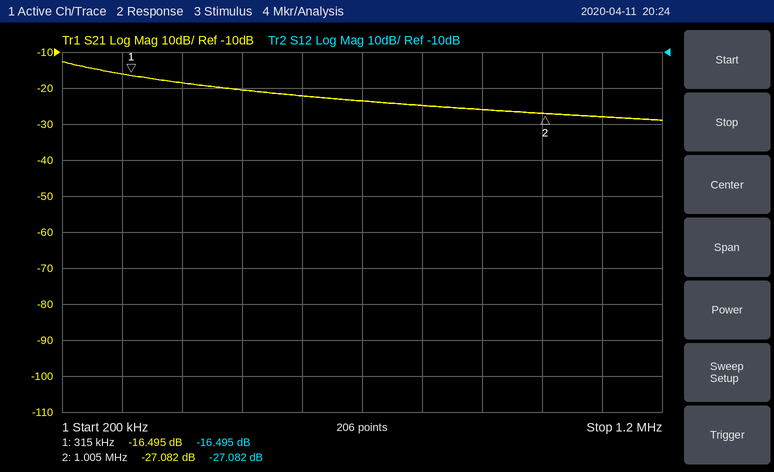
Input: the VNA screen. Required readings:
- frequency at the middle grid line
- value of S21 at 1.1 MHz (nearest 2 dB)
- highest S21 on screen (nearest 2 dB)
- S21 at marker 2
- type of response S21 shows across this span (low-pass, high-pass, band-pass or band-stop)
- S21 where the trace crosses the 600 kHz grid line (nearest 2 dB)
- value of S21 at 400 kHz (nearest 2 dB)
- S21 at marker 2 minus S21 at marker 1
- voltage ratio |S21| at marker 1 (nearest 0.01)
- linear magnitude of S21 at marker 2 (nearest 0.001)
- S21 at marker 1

700 kHz
-28 dB
-12 dB
-27.082 dB
low-pass
-22 dB
-18 dB
-10.587 dB
0.15
0.044
-16.495 dB
